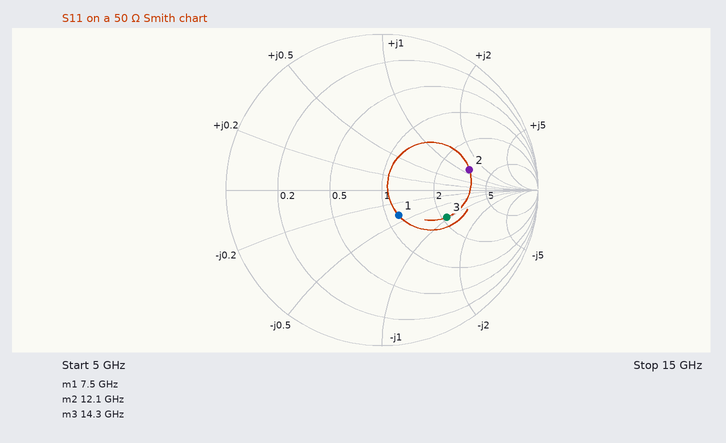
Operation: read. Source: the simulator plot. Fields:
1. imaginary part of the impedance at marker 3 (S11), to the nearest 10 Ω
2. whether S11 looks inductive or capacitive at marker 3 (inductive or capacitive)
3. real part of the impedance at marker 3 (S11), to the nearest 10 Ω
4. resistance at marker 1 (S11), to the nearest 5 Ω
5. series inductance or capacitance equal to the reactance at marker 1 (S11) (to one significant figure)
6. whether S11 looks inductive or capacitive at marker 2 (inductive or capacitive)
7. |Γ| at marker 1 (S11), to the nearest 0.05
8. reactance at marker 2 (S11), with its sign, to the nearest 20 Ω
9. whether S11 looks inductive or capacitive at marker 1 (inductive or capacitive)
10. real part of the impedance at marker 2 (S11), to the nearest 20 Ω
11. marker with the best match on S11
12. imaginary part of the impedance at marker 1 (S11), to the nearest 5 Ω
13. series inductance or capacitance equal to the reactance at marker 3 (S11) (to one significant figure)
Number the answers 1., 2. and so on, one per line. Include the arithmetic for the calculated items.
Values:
1. -50 Ω
2. capacitive
3. 110 Ω
4. 60 Ω
5. C = 1/(2π × 7.5 GHz × 20 Ω) ≈ 1 pF
6. inductive
7. 0.20
8. +60 Ω
9. capacitive
10. 160 Ω
11. marker 1
12. -20 Ω
13. C = 1/(2π × 14.3 GHz × 50 Ω) ≈ 223 fF, so 200 fF to one significant figure
